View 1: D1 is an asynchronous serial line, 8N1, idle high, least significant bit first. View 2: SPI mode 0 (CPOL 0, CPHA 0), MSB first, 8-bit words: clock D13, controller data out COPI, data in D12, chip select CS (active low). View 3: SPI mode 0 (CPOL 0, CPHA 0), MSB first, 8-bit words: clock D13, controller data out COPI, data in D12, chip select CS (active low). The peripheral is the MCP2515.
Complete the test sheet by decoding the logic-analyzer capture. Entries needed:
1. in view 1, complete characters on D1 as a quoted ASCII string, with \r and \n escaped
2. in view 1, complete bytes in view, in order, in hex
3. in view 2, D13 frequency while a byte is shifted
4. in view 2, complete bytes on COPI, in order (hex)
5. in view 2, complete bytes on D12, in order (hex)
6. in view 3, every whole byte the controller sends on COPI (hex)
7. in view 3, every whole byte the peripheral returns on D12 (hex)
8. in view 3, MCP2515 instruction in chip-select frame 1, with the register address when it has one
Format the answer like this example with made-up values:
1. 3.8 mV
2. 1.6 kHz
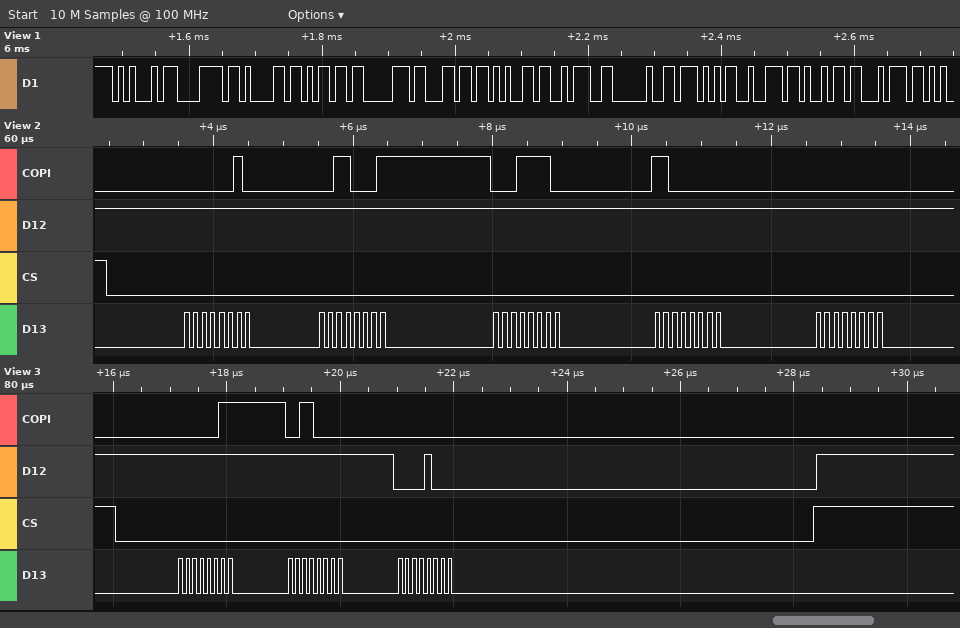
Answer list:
1. "Example: Writ"
2. 45 78 61 6D 70 6C 65 3A 20 57 72 69 74
3. 8 MHz
4. 02 31 1E C0 00
5. FF FF FF FF FF
6. 03 30 00
7. FF FF 08
8. READ 0x30
